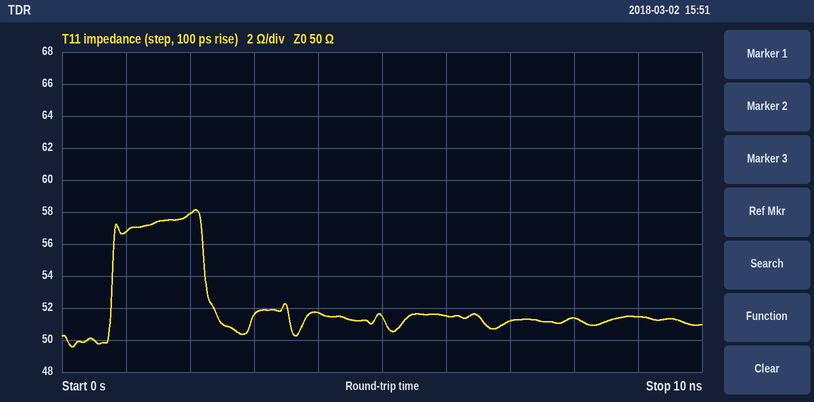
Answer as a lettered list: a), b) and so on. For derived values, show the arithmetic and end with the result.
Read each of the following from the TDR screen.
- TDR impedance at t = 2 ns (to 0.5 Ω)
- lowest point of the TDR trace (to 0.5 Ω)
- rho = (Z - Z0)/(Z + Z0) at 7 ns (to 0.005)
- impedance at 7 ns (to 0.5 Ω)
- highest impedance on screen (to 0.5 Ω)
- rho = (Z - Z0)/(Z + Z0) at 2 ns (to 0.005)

a) 58.0 Ω
b) 49.5 Ω
c) (51 − 50)/(51 + 50) ≈ +0.010
d) 51.0 Ω
e) 58.0 Ω
f) (58 − 50)/(58 + 50) ≈ +0.0741, so +0.075 to the nearest 0.005
